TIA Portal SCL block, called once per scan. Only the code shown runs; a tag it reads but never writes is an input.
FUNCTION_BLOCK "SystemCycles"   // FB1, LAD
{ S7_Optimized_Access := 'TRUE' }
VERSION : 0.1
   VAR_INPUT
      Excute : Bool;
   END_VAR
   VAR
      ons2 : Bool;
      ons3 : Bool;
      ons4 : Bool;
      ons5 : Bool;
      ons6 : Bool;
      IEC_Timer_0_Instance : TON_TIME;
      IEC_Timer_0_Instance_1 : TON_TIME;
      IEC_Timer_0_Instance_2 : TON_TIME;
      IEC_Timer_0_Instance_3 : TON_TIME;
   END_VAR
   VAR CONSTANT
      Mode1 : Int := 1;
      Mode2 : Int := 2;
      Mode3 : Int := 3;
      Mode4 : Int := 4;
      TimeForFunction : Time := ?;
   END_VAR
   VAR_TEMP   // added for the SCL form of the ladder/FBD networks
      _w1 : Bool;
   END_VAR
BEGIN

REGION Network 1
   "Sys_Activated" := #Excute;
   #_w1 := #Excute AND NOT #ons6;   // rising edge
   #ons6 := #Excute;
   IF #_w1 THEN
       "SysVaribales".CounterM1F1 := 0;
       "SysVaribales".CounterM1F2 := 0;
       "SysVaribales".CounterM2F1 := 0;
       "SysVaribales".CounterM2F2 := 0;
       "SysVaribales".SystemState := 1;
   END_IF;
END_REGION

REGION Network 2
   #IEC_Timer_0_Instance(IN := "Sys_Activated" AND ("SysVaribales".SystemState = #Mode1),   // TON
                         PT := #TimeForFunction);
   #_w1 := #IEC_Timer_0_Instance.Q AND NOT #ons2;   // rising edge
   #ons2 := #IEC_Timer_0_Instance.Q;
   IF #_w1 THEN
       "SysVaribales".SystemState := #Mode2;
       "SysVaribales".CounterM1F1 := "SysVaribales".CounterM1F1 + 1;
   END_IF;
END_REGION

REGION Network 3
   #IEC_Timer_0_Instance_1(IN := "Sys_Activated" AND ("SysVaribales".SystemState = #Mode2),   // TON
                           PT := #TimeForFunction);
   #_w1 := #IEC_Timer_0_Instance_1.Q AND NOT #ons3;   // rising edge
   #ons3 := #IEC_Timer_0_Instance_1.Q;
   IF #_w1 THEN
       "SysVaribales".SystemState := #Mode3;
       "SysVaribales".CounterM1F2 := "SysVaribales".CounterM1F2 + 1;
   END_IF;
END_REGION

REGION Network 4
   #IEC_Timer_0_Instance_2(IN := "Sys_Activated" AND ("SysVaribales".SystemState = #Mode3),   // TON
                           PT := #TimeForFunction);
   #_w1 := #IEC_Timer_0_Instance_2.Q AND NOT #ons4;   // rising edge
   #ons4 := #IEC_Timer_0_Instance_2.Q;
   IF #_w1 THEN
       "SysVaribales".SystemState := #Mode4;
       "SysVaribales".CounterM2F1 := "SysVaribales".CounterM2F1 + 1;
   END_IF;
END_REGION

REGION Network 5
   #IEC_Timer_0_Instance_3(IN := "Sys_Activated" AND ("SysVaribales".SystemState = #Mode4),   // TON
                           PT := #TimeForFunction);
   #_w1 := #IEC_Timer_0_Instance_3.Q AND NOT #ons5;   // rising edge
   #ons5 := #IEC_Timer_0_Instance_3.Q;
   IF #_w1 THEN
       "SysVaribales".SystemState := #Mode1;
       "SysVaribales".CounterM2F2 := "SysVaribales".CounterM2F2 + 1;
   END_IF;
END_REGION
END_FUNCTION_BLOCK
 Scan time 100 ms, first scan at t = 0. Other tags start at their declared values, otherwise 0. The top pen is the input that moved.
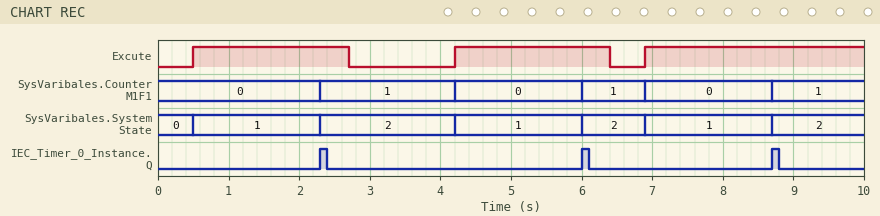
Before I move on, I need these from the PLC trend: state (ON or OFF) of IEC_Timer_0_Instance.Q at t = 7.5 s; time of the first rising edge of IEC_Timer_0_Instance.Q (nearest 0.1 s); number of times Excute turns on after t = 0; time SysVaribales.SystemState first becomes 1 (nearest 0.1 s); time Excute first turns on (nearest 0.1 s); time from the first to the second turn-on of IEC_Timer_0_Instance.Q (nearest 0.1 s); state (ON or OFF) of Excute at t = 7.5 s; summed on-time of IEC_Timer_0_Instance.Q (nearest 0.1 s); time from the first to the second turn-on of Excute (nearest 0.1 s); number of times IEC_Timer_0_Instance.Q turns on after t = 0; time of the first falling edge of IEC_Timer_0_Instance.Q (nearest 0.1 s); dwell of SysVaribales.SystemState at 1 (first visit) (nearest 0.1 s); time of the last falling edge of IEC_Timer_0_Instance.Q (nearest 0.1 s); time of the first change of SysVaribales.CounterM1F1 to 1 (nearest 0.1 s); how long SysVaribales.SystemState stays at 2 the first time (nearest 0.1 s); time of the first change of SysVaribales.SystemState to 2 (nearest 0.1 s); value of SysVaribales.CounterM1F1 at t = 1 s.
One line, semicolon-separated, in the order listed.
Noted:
OFF; 2.3 s; 3; 0.5 s; 0.5 s; 3.7 s; ON; 0.3 s; 3.7 s; 3; 2.4 s; 1.8 s; 8.8 s; 2.3 s; 1.9 s; 2.3 s; 0
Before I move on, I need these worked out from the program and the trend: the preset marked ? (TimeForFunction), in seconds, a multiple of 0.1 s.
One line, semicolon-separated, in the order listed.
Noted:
1.8 s
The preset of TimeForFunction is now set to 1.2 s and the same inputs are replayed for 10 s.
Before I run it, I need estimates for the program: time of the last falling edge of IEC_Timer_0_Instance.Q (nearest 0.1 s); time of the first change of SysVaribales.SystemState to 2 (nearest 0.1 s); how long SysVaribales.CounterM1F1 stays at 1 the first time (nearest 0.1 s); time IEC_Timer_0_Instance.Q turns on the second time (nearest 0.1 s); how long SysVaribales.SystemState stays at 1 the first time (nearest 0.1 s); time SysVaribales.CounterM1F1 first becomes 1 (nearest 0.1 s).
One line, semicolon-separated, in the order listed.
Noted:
8.2 s; 1.7 s; 2.5 s; 5.4 s; 1.2 s; 1.7 s
